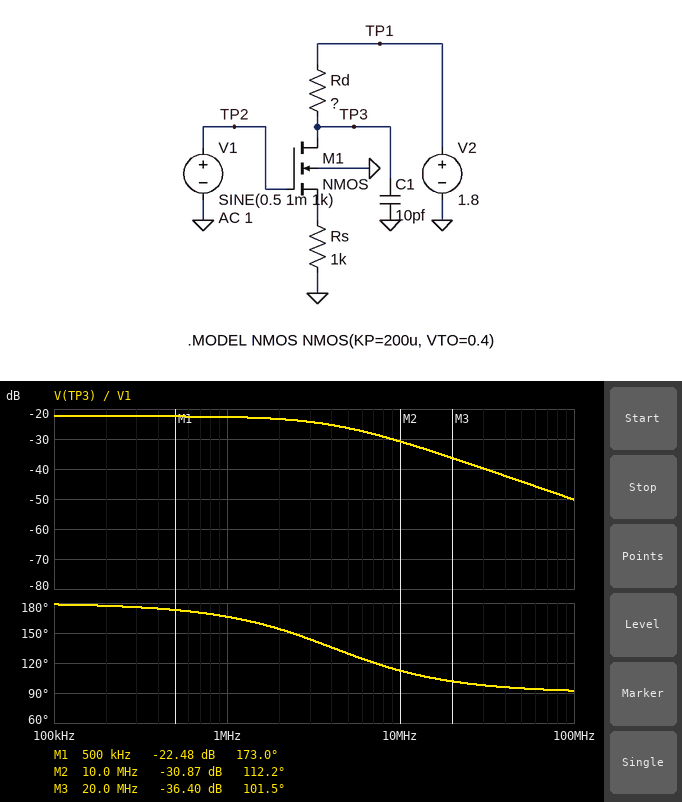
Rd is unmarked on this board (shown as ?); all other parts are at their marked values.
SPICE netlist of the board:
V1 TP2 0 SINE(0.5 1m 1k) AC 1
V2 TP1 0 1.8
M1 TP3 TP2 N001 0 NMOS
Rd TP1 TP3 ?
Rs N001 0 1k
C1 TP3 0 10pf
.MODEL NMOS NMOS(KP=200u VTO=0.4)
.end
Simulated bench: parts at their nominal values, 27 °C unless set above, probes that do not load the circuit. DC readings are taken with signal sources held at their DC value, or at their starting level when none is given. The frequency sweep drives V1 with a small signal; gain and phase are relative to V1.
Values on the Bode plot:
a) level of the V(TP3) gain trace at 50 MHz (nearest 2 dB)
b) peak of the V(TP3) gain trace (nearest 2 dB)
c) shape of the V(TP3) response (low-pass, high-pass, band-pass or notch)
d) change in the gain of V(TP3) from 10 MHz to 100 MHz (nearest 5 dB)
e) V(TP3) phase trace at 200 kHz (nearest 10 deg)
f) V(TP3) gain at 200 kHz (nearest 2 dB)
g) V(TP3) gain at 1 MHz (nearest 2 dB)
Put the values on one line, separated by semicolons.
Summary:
-44 dB; -22 dB; low-pass; -20 dB; 180 deg; -22 dB; -22 dB
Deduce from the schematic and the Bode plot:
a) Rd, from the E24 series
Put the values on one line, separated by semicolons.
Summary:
3.9 kΩ
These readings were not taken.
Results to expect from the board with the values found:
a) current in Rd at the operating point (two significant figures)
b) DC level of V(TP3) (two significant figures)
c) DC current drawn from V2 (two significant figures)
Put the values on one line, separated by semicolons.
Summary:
980 nA; 1.8 V; 980 nA
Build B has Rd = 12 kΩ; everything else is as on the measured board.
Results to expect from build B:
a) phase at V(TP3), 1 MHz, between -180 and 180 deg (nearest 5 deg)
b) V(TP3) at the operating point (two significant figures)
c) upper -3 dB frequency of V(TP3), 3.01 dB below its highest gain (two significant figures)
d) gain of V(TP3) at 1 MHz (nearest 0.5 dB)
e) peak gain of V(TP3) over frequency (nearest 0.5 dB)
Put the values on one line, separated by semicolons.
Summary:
145 deg; 1.8 V; 1.3 MHz; -14.5 dB; -12.5 dB
